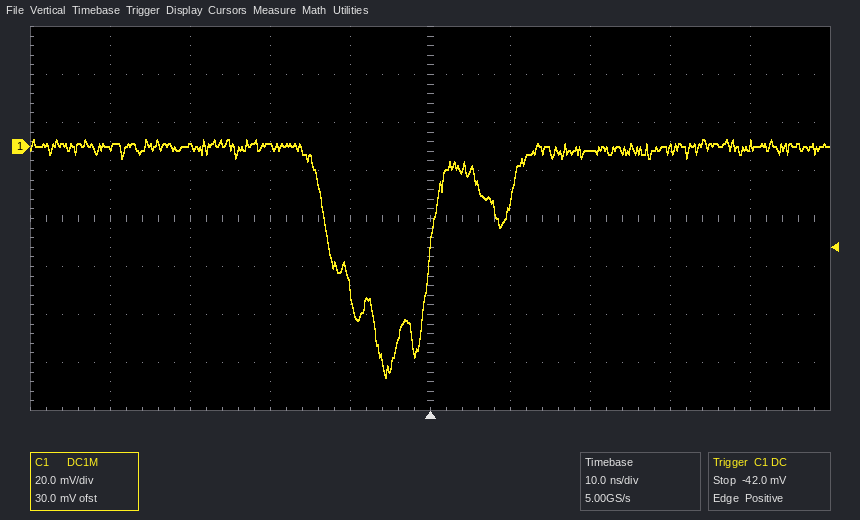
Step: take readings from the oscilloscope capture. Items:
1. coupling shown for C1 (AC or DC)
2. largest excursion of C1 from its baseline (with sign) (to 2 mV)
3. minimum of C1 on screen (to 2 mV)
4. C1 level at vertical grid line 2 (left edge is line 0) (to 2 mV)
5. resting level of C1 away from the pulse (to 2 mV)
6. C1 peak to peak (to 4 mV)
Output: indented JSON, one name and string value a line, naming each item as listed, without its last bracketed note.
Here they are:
{
  "coupling shown for C1": "DC",
  "largest excursion of C1 from its baseline (with sign)": "-96 mV",
  "minimum of C1 on screen": "-96 mV",
  "C1 level at vertical grid line 2 (left edge is line 0)": "0 mV",
  "resting level of C1 away from the pulse": "0 mV",
  "C1 peak to peak": "100 mV"
}
